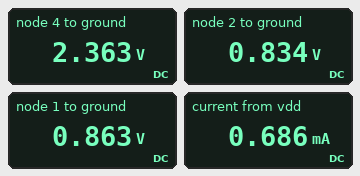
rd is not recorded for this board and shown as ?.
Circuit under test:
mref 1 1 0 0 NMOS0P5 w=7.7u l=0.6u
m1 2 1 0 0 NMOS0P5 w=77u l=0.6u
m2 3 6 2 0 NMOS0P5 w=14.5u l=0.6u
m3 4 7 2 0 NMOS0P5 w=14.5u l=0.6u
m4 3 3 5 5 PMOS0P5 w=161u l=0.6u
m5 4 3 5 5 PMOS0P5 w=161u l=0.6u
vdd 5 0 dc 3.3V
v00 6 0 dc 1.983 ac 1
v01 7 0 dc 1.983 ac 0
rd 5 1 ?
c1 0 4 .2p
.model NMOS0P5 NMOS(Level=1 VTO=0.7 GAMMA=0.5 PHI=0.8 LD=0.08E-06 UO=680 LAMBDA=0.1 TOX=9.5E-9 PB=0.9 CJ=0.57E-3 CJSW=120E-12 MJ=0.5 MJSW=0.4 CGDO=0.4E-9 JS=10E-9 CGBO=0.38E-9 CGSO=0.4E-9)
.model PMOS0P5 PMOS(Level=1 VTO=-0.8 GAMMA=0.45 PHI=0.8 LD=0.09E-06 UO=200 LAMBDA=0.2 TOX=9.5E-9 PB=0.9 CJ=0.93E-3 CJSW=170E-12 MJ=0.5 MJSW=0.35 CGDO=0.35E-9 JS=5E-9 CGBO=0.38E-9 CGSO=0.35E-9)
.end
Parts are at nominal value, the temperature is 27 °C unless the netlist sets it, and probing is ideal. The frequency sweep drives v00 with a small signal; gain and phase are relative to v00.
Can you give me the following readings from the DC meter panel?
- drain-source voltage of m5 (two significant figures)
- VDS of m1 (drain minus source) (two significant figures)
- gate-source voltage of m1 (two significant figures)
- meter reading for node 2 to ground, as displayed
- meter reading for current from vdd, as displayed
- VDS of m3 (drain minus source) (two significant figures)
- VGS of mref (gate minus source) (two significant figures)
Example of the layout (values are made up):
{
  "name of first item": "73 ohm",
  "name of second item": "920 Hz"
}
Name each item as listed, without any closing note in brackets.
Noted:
{
  "drain-source voltage of m5": "-940 mV",
  "VDS of m1 (drain minus source)": "830 mV",
  "gate-source voltage of m1": "860 mV",
  "meter reading for node 2 to ground, as displayed": "0.834 V",
  "meter reading for current from vdd, as displayed": "0.686 mA",
  "VDS of m3 (drain minus source)": "1.5 V",
  "VGS of mref (gate minus source)": "860 mV"
}
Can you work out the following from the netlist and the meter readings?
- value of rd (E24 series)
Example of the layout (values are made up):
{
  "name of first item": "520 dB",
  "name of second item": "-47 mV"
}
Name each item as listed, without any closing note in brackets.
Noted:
{
  "value of rd": "39 kΩ"
}
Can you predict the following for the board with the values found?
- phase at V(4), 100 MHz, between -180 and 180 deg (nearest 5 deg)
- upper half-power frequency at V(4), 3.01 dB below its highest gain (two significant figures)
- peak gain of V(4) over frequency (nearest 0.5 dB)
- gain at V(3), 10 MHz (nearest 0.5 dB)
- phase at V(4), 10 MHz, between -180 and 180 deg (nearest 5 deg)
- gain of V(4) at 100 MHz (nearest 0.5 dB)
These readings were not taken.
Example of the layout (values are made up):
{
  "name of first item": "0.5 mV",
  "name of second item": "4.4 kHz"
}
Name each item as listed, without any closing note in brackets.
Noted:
{
  "phase at V(4), 100 MHz, between -180 and 180 deg": "-70 deg",
  "upper half-power frequency at V(4), 3.01 dB below its highest gain": "40 MHz",
  "peak gain of V(4) over frequency": "29.5 dB",
  "gain at V(3), 10 MHz": "-15.0 dB",
  "phase at V(4), 10 MHz, between -180 and 180 deg": "-15 deg",
  "gain of V(4) at 100 MHz": "21.0 dB"
}
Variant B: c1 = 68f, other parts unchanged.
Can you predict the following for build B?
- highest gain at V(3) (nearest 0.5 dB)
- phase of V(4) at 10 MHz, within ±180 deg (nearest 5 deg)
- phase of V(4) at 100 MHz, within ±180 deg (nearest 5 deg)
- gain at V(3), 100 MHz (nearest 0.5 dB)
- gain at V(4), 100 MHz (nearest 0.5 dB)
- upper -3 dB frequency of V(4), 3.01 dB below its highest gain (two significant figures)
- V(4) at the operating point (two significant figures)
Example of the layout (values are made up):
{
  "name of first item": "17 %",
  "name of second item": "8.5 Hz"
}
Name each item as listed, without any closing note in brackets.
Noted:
{
  "highest gain at V(3)": "-15.0 dB",
  "phase of V(4) at 10 MHz, within ±180 deg": "-10 deg",
  "phase of V(4) at 100 MHz, within ±180 deg": "-55 deg",
  "gain at V(3), 100 MHz": "-17.5 dB",
  "gain at V(4), 100 MHz": "24.5 dB",
  "upper -3 dB frequency of V(4), 3.01 dB below its highest gain": "68 MHz",
  "V(4) at the operating point": "2.4 V"
}
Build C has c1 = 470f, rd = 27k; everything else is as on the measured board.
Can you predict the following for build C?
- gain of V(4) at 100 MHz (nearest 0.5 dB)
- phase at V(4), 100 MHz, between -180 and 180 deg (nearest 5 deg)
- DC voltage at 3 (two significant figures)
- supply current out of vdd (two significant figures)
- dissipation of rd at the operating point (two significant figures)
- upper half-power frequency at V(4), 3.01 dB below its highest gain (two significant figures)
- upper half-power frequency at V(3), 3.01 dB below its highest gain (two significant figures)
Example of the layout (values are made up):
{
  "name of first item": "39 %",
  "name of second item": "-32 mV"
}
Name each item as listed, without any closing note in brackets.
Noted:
{
  "gain of V(4) at 100 MHz": "17.5 dB",
  "phase at V(4), 100 MHz, between -180 and 180 deg": "-75 deg",
  "DC voltage at 3": "2.3 V",
  "supply current out of vdd": "970 µA",
  "dissipation of rd at the operating point": "210 µW",
  "upper half-power frequency at V(4), 3.01 dB below its highest gain": "30 MHz",
  "upper half-power frequency at V(3), 3.01 dB below its highest gain": "2.6 GHz"
}
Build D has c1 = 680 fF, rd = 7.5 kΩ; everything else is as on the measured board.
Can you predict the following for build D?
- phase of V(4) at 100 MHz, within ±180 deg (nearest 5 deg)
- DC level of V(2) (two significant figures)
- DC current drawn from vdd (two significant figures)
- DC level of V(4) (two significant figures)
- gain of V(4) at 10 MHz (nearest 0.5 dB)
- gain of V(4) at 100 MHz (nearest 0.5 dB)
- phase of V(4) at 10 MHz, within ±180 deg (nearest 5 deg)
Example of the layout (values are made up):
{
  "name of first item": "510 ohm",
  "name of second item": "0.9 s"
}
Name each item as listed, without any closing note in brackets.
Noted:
{
  "phase of V(4) at 100 MHz, within ±180 deg": "-55 deg",
  "DC level of V(2)": "590 mV",
  "DC current drawn from vdd": "3.2 mA",
  "DC level of V(4)": "2.2 V",
  "gain of V(4) at 10 MHz": "23.0 dB",
  "gain of V(4) at 100 MHz": "18.5 dB",
  "phase of V(4) at 10 MHz, within ±180 deg": "-10 deg"
}
